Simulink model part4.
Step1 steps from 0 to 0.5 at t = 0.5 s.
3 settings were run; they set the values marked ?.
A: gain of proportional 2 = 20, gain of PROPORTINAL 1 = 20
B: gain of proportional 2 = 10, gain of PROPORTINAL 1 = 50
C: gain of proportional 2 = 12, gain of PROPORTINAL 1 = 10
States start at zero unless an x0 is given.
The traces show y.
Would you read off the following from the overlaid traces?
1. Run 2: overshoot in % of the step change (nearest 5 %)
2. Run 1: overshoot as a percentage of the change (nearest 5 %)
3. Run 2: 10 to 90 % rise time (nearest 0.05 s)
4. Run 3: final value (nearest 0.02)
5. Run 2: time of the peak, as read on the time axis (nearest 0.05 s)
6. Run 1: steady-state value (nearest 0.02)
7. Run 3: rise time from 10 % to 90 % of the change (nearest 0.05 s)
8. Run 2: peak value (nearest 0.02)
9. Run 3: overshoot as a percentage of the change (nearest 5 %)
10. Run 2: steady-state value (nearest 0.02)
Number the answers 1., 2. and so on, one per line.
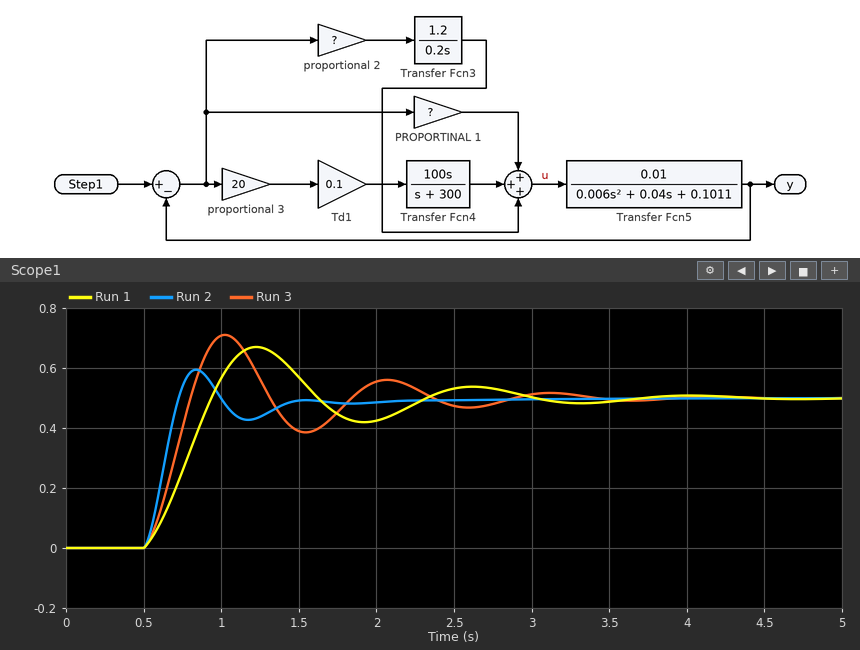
1. 20 %
2. 35 %
3. 0.15 s
4. 0.50
5. 0.85 s
6. 0.50
7. 0.20 s
8. 0.60
9. 40 %
10. 0.50
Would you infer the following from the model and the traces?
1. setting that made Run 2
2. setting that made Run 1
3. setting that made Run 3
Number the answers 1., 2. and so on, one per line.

1. B
2. C
3. A
